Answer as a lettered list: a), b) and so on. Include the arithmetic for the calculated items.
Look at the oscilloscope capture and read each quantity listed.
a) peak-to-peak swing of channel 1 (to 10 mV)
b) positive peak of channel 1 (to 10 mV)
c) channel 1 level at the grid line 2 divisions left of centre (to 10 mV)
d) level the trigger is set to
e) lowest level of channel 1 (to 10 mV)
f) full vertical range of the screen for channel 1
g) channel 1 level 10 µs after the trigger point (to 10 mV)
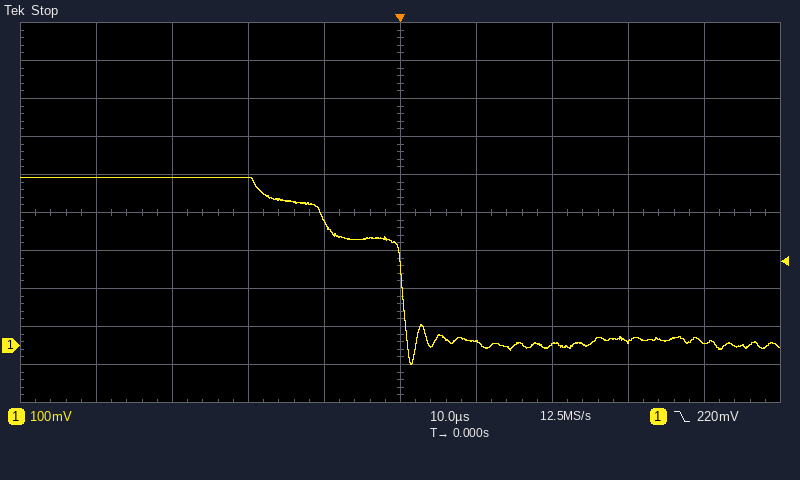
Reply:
a) 440 mV − (-50 mV) = 490 mV
b) 440 mV
c) 440 mV
d) 220 mV
e) -50 mV
f) 1 V
g) 10 mV
